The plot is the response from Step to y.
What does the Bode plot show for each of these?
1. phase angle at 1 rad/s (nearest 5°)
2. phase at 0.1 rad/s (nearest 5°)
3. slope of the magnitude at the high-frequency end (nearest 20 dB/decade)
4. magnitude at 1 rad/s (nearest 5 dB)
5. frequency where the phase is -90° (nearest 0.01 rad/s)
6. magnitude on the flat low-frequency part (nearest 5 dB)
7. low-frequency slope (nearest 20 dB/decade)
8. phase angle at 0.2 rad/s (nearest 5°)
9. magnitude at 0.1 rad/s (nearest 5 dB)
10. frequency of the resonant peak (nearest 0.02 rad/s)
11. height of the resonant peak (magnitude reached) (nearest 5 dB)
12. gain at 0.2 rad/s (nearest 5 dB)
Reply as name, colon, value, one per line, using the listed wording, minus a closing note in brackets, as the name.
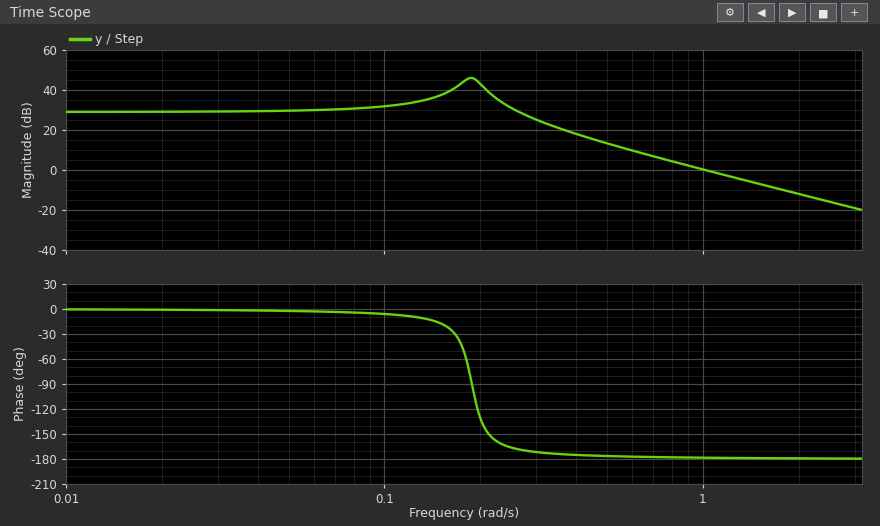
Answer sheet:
phase angle at 1 rad/s: -180°
phase at 0.1 rad/s: -5°
slope of the magnitude at the high-frequency end: -40 dB/decade
magnitude at 1 rad/s: 0 dB
frequency where the phase is -90°: 0.19 rad/s
magnitude on the flat low-frequency part: 30 dB
low-frequency slope: 0 dB/decade
phase angle at 0.2 rad/s: -130°
magnitude at 0.1 rad/s: 30 dB
frequency of the resonant peak: 0.18 rad/s
height of the resonant peak (magnitude reached): 45 dB
gain at 0.2 rad/s: 45 dB
